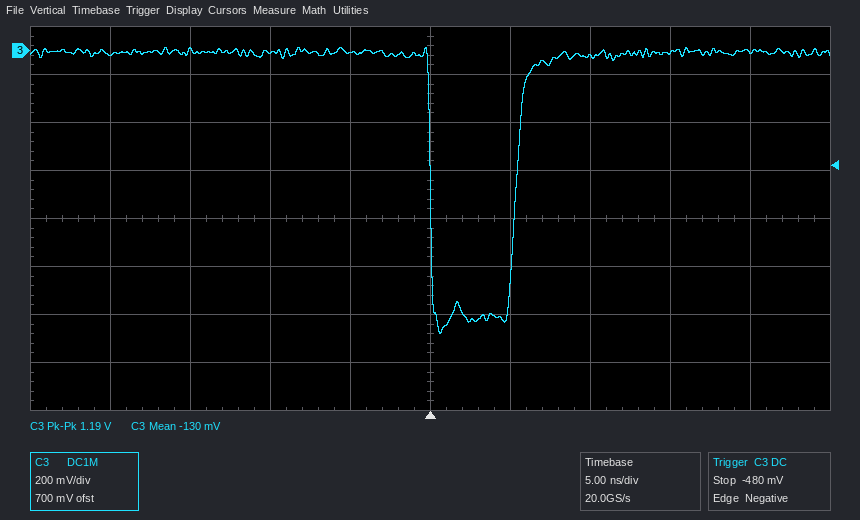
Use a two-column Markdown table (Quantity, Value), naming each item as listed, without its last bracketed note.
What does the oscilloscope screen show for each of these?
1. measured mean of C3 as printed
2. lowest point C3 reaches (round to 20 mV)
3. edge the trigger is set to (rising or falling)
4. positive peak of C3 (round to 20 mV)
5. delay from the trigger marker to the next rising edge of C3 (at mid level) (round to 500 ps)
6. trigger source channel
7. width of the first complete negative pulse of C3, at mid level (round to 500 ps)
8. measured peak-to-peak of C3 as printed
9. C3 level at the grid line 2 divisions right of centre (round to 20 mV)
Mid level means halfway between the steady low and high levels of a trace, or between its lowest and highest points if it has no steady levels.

| Quantity | Value |
|---|---|
| measured mean of C3 as printed | -130 mV |
| lowest point C3 reaches | -1.18 V |
| edge the trigger is set to | falling |
| positive peak of C3 | 20 mV |
| delay from the trigger marker to the next rising edge of C3 (at mid level) | 5.5 ns |
| trigger source channel | C3 |
| width of the first complete negative pulse of C3, at mid level | 5.5 ns |
| measured peak-to-peak of C3 as printed | 1.19 V |
| C3 level at the grid line 2 divisions right of centre | -20 mV |
